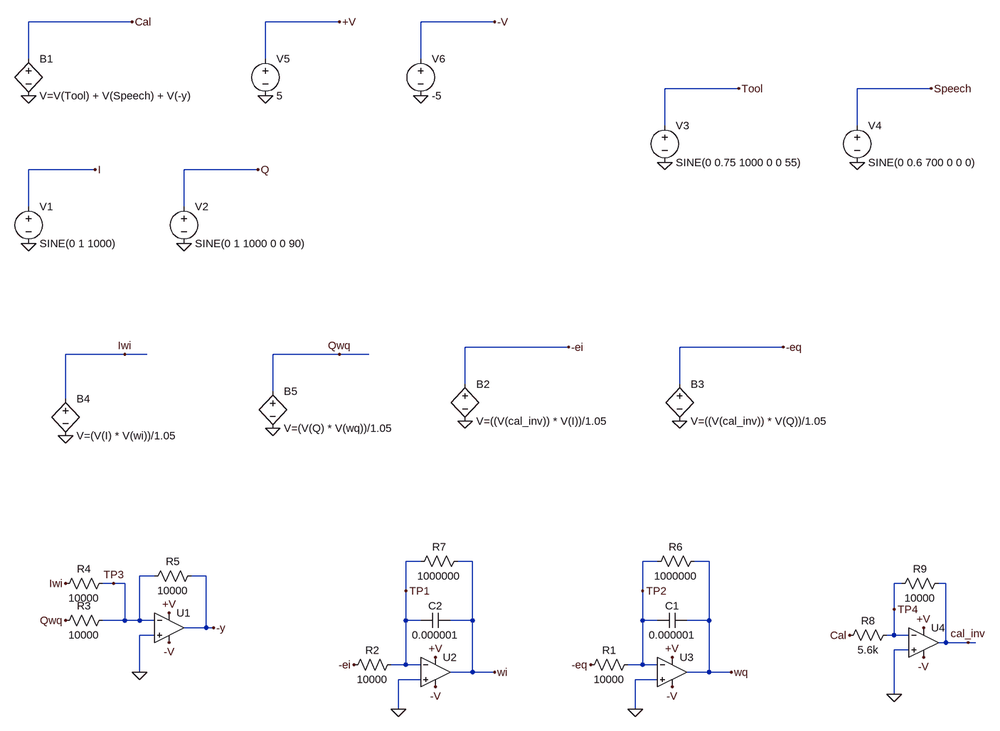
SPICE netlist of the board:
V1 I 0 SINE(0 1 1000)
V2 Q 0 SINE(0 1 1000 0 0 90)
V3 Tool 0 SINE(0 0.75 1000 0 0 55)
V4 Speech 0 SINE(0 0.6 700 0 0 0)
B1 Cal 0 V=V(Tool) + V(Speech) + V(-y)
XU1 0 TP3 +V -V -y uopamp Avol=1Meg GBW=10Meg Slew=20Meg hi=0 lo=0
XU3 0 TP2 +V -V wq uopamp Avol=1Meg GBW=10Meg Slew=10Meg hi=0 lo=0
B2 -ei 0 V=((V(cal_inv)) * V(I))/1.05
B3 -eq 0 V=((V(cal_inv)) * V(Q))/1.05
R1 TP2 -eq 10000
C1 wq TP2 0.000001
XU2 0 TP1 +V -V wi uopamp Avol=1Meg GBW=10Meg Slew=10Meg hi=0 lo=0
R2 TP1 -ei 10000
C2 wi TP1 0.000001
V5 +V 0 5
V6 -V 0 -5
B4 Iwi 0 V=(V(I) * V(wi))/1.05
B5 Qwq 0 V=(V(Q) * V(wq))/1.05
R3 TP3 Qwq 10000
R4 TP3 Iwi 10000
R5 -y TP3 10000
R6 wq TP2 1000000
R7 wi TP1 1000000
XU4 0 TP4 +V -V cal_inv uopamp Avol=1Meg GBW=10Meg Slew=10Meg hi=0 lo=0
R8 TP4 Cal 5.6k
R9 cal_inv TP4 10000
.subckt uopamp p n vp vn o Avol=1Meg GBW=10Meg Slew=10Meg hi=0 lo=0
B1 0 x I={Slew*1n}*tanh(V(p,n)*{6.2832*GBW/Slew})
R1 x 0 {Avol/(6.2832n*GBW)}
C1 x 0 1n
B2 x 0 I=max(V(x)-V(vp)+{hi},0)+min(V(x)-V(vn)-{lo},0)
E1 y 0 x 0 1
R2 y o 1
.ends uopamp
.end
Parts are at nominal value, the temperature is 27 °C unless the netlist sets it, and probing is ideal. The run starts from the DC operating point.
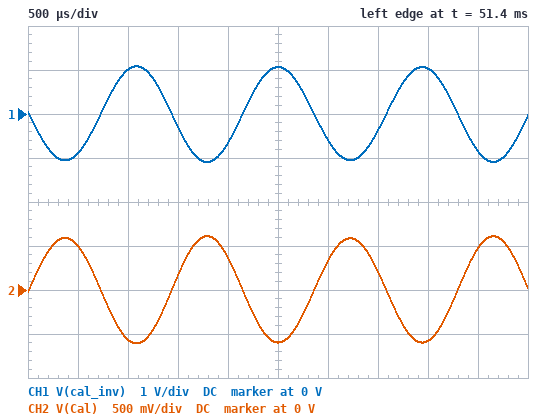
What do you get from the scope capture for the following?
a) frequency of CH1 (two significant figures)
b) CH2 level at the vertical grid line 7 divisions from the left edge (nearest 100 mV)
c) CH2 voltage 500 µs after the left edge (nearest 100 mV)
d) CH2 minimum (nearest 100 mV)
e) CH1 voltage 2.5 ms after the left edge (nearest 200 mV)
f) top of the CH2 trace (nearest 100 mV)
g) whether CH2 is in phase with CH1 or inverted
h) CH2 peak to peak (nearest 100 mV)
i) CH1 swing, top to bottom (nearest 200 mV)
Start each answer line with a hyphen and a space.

- 700 Hz
- 200 mV
- 500 mV
- -600 mV
- 1.0 V
- 600 mV
- inverted
- 1.2 V
- 2.2 V
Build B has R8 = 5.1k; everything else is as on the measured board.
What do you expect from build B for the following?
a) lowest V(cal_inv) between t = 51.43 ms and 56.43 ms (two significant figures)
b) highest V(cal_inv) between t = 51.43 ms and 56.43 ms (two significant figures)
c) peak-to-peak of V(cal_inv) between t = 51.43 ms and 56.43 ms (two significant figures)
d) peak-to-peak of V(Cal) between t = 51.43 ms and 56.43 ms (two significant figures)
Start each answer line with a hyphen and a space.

- -1.2 V
- 1.2 V
- 2.4 V
- 1.2 V
